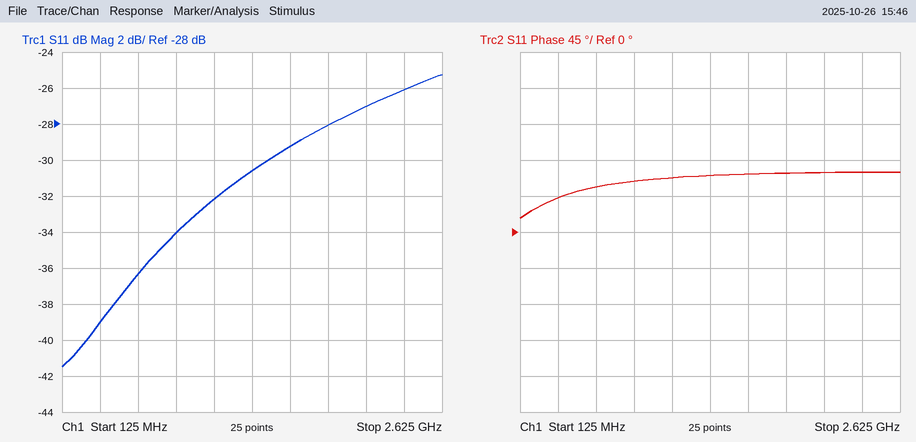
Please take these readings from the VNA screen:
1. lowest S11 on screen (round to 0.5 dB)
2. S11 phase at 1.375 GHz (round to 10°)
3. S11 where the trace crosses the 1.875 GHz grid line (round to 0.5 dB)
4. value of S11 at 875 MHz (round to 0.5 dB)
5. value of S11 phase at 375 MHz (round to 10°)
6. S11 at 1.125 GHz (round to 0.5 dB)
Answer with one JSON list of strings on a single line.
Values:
["-41.5 dB", "70°", "-28.0 dB", "-34.0 dB", "40°", "-32.0 dB"]
